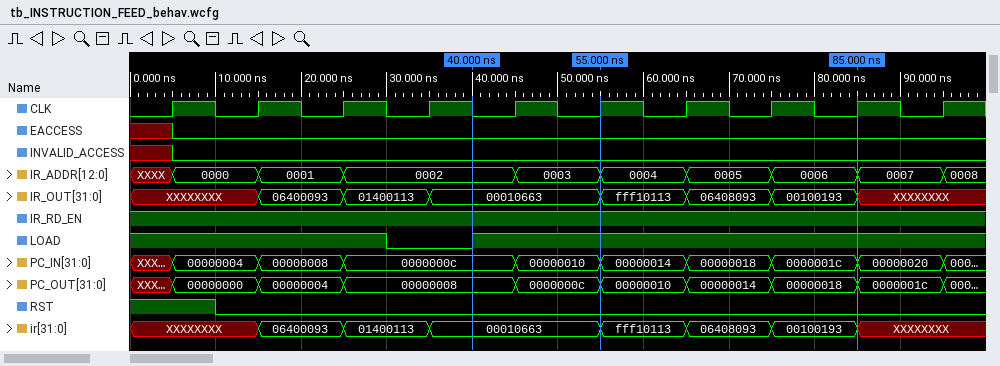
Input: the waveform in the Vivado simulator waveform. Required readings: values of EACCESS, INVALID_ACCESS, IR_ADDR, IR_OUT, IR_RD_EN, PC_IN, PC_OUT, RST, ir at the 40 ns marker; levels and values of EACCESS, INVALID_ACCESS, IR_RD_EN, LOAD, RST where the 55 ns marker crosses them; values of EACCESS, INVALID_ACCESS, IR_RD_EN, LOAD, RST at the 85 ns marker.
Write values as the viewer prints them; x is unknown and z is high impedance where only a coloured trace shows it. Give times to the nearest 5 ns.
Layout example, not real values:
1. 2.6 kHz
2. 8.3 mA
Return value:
1. EACCESS=0, INVALID_ACCESS=0, IR_ADDR=0002, IR_OUT=00010663, IR_RD_EN=1, PC_IN=0000000c, PC_OUT=00000008, RST=0, ir=00010663
2. EACCESS=0, INVALID_ACCESS=0, IR_RD_EN=1, LOAD=1, RST=0
3. EACCESS=0, INVALID_ACCESS=0, IR_RD_EN=1, LOAD=1, RST=0
